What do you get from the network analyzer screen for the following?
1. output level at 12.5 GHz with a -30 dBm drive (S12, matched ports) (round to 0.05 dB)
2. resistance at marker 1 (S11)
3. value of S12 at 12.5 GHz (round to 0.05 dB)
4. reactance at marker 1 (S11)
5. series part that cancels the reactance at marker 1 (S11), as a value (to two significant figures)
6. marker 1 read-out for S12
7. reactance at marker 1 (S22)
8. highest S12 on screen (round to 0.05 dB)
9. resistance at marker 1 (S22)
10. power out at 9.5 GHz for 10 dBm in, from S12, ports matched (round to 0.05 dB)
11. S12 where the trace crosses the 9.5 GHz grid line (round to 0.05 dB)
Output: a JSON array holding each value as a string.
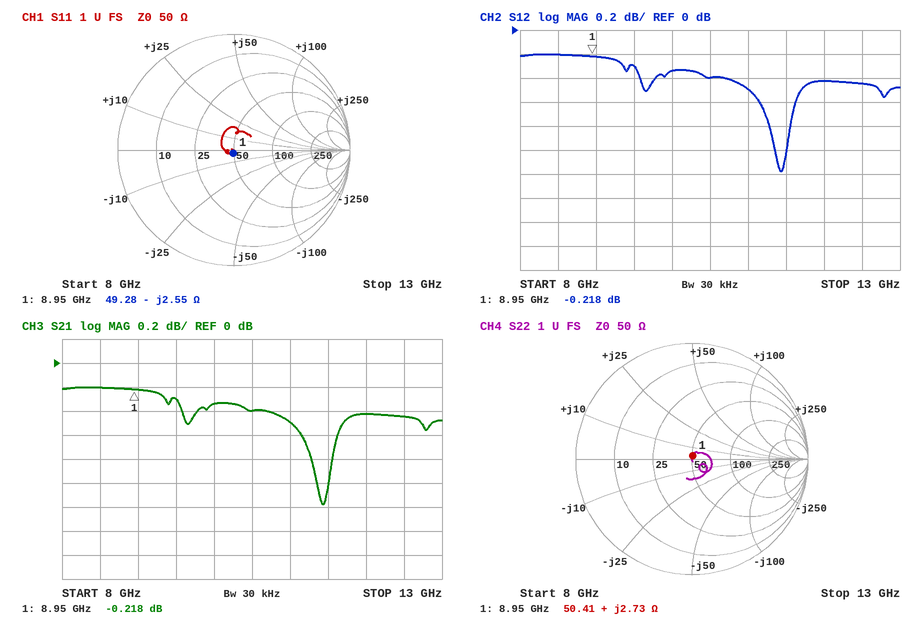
["-30.45 dBm", "49.28 Ω", "-0.45 dB", "-2.55 Ω", "45 pH", "-0.218 dB", "+2.73 Ω", "-0.20 dB", "50.41 Ω", "9.70 dBm", "-0.30 dB"]
